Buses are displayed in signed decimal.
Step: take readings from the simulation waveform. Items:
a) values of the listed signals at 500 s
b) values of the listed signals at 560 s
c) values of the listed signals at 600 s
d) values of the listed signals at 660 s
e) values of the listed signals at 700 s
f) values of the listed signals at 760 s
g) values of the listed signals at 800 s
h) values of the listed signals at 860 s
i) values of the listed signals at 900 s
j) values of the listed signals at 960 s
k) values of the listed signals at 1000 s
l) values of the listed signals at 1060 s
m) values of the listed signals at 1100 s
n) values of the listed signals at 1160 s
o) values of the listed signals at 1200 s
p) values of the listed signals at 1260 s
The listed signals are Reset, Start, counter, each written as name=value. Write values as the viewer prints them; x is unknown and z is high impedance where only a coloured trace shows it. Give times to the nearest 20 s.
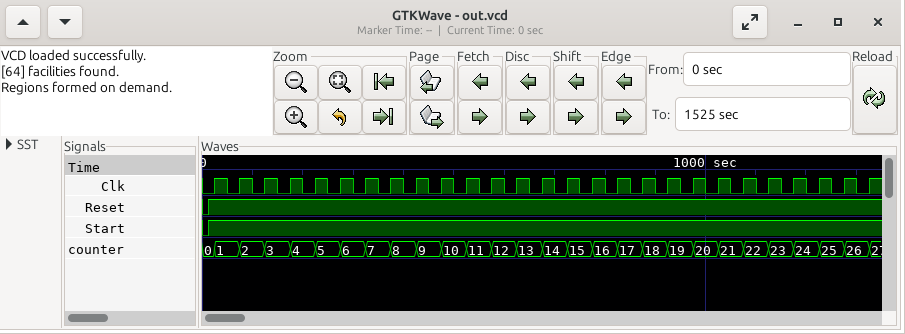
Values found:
Reset=1, Start=1, counter=10
Reset=1, Start=1, counter=11
Reset=1, Start=1, counter=12
Reset=1, Start=1, counter=13
Reset=1, Start=1, counter=14
Reset=1, Start=1, counter=15
Reset=1, Start=1, counter=16
Reset=1, Start=1, counter=17
Reset=1, Start=1, counter=18
Reset=1, Start=1, counter=19
Reset=1, Start=1, counter=20
Reset=1, Start=1, counter=21
Reset=1, Start=1, counter=22
Reset=1, Start=1, counter=23
Reset=1, Start=1, counter=24
Reset=1, Start=1, counter=25
